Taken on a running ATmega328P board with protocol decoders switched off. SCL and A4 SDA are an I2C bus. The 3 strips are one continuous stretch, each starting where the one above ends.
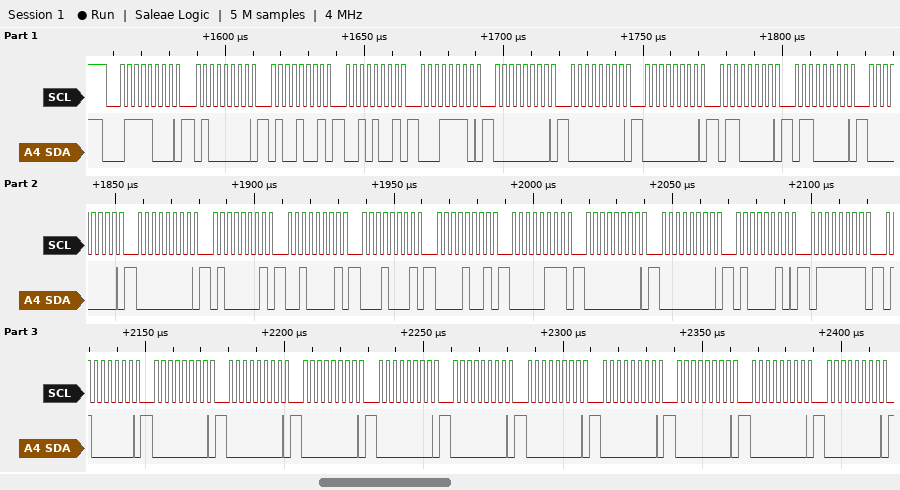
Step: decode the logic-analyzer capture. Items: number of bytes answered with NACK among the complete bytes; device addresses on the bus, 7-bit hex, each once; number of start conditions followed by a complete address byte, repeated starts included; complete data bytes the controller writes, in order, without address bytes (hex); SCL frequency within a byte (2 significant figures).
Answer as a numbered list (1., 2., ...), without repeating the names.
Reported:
1. 0
2. 0x3C
3. 1
4. 40 49 29 1E 00 00 00 60 60 00 00 41 21 11 09 07 00 00 42 7F 40 00 00 00 00 00 00 00 00 00 00
5. 400 kHz
